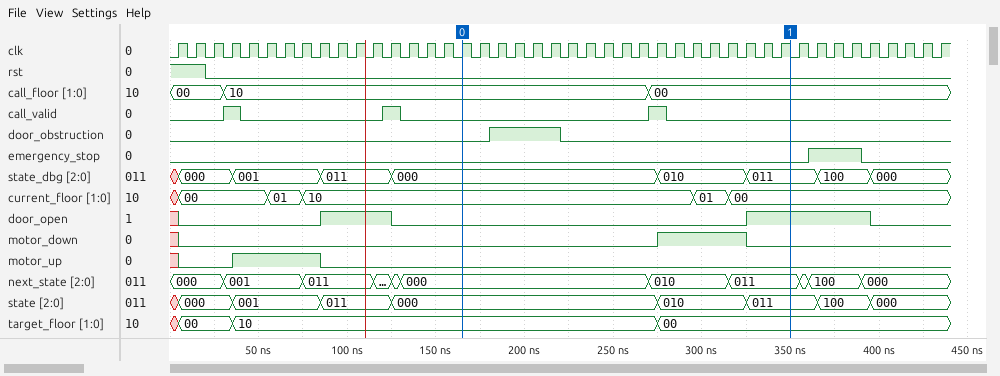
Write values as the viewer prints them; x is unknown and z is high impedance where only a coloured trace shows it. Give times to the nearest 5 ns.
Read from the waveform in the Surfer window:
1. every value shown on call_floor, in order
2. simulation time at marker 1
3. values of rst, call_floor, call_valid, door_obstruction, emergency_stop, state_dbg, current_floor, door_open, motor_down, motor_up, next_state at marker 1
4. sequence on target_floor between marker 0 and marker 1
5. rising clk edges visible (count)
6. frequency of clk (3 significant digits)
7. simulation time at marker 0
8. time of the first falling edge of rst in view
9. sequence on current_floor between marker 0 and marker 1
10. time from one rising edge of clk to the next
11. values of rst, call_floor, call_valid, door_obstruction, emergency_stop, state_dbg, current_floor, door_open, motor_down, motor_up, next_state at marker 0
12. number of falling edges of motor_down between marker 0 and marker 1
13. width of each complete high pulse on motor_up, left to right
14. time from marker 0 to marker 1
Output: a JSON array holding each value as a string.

["00, 10, 00", "350 ns", "rst=0, call_floor=00, call_valid=0, door_obstruction=0, emergency_stop=0, state_dbg=011, current_floor=00, door_open=1, motor_down=0, motor_up=0, next_state=011", "10, 00", "44", "100 MHz", "165 ns", "20 ns", "10, 01, 00", "10 ns", "rst=0, call_floor=10, call_valid=0, door_obstruction=0, emergency_stop=0, state_dbg=000, current_floor=10, door_open=0, motor_down=0, motor_up=0, next_state=000", "1", "50 ns", "185 ns"]
